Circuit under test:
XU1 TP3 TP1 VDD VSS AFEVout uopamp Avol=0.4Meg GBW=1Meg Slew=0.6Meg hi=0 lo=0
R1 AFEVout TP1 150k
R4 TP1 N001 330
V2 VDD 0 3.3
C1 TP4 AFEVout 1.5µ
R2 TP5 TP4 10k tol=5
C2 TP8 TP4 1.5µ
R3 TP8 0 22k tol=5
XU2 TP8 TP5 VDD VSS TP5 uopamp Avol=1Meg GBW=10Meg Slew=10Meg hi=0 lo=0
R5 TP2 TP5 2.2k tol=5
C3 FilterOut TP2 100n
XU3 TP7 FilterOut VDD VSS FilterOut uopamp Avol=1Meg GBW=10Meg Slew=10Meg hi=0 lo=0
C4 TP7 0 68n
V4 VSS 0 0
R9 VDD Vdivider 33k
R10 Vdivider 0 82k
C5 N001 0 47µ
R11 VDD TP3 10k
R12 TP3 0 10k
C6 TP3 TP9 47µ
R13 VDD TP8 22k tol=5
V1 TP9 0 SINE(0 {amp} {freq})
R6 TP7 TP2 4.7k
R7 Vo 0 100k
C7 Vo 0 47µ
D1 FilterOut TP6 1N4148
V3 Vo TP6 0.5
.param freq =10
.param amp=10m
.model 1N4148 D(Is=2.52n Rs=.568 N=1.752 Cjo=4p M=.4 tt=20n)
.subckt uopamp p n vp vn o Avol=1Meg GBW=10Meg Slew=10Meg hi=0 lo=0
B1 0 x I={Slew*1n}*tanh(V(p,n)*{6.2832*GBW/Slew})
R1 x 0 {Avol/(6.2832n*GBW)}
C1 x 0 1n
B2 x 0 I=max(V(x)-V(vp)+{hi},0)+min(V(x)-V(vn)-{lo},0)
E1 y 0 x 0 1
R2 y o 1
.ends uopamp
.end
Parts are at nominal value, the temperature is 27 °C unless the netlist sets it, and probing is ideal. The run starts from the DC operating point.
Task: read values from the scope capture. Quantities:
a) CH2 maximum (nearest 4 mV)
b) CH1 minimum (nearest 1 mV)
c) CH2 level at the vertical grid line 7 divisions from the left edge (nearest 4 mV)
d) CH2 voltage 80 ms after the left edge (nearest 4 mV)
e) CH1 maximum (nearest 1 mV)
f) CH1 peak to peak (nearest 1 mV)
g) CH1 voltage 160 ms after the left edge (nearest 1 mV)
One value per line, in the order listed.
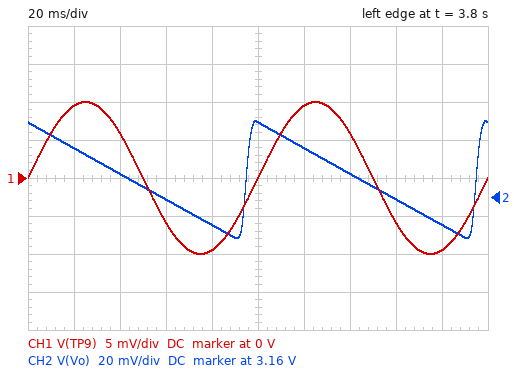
3.200 V
-10 mV
3.172 V
3.144 V
10 mV
20 mV
-6 mV
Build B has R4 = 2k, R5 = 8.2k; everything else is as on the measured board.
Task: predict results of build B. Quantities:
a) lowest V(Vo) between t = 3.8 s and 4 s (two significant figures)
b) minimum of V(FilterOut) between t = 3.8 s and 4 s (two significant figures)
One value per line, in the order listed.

2.0 V
1.3 V
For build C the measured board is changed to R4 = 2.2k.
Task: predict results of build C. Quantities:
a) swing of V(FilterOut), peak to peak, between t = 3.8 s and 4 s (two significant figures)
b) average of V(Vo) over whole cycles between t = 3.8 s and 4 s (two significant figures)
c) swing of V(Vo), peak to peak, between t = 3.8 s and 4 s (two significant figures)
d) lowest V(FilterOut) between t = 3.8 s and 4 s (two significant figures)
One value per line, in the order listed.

710 mV
2.0 V
31 mV
1.3 V
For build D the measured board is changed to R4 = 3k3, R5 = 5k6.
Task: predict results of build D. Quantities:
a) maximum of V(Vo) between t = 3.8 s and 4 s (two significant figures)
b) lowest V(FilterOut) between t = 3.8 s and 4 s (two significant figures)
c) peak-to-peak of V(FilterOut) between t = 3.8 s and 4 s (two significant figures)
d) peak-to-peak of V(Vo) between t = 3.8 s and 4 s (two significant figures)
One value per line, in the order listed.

1.9 V
1.4 V
480 mV
27 mV
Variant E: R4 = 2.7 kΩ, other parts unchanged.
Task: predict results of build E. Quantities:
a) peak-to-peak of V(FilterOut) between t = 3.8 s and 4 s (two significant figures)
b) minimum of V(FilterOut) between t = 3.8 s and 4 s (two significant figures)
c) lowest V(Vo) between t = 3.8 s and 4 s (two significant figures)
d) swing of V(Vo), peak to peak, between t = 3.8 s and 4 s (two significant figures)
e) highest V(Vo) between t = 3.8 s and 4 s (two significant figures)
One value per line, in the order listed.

580 mV
1.4 V
1.9 V
29 mV
2.0 V
